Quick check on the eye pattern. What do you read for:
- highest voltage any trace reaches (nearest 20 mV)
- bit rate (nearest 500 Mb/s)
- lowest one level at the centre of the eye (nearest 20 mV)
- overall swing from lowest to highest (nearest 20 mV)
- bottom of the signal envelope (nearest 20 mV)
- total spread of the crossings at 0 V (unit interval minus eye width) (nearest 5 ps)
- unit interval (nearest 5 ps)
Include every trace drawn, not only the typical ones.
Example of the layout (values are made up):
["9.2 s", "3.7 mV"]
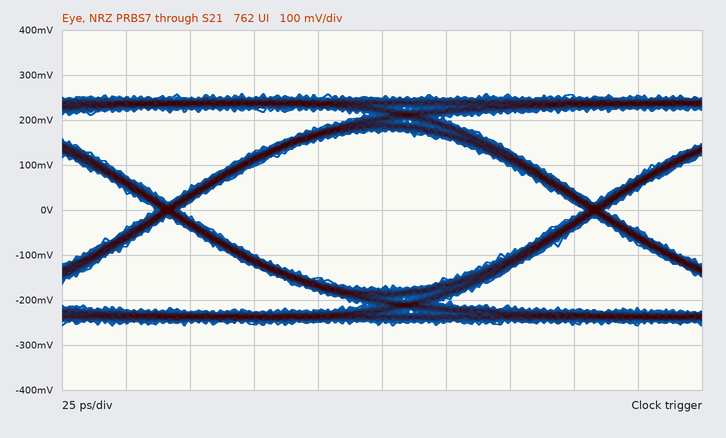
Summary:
["260 mV", "6.0 Gb/s", "180 mV", "520 mV", "-260 mV", "10 ps", "165 ps"]
